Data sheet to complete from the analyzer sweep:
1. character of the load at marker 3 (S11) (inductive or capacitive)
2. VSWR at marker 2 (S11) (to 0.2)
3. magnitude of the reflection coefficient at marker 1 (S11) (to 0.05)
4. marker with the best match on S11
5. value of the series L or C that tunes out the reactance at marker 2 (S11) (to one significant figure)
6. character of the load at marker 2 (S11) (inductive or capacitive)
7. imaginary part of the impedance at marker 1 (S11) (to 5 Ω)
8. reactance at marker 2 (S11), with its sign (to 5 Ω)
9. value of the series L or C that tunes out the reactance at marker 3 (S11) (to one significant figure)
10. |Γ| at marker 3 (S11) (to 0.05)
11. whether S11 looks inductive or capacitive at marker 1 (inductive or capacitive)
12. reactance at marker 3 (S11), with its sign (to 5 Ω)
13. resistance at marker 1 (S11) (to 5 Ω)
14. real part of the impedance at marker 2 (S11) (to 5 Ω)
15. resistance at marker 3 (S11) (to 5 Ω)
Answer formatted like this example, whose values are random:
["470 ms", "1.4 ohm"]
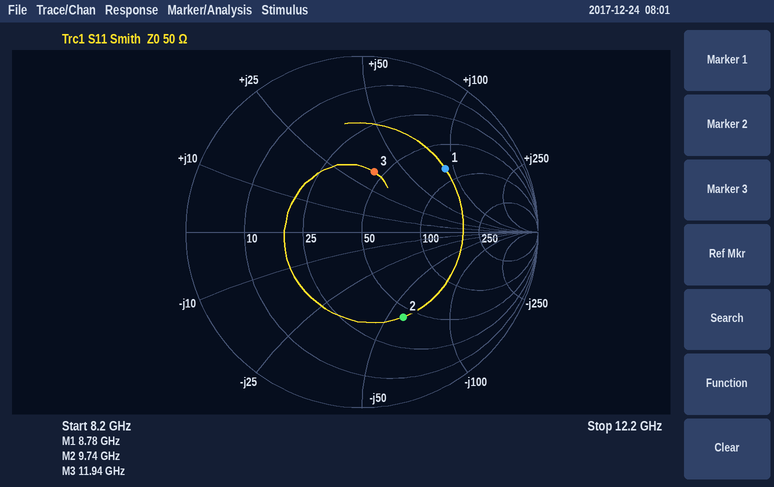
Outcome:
["inductive", "3.4", "0.60", "marker 3", "1.0 nH", "capacitive", "+90 Ω", "-60 Ω", "400 fF", "0.35", "inductive", "+35 Ω", "80 Ω", "45 Ω", "45 Ω"]
